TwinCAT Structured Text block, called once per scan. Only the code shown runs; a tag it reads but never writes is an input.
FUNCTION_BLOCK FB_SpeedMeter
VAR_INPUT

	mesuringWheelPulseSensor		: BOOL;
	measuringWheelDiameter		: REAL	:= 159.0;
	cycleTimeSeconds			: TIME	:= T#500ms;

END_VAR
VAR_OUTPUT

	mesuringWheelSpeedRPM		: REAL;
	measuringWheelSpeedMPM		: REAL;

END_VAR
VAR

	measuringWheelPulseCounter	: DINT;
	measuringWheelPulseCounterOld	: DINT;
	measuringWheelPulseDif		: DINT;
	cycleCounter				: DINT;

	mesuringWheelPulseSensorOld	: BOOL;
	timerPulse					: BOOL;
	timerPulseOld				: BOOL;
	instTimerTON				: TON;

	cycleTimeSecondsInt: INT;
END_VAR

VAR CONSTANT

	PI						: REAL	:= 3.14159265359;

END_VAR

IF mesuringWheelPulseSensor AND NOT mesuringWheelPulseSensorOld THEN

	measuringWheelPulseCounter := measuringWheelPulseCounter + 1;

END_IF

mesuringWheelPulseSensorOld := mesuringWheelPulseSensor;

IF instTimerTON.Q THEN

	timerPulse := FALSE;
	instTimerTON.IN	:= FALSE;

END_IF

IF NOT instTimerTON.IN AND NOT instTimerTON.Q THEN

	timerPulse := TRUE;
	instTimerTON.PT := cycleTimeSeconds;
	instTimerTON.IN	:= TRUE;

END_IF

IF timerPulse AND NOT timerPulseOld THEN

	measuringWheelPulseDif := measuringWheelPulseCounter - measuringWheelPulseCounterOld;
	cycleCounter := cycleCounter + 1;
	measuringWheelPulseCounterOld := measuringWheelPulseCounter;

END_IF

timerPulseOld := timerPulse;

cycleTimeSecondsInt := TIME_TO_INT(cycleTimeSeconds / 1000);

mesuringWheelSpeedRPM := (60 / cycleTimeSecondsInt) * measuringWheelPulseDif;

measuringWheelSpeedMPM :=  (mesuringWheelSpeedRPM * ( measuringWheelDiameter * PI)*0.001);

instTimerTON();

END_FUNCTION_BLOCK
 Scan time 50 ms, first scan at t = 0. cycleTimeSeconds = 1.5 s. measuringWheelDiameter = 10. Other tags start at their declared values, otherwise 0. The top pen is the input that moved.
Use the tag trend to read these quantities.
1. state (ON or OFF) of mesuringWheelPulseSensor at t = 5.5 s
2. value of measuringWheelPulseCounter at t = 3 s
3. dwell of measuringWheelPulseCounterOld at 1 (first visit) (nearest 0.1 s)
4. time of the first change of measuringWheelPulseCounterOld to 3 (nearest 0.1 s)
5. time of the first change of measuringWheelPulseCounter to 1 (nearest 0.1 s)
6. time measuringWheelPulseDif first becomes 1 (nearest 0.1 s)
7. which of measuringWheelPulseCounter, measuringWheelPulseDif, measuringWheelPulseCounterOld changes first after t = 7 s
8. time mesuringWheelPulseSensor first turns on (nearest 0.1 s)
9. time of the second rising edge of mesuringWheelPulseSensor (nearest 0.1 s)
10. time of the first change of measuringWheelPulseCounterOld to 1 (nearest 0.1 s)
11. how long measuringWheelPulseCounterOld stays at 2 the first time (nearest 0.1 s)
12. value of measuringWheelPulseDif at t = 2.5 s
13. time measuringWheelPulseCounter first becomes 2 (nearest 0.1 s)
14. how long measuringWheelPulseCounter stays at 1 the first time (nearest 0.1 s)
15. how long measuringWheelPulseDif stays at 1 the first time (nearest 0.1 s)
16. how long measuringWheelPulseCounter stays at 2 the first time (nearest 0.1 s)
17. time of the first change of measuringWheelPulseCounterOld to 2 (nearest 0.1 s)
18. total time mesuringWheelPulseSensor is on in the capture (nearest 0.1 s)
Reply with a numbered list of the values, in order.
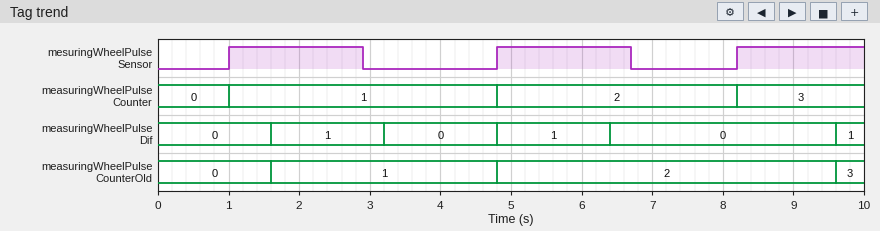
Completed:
1. ON
2. 1
3. 3.2 s
4. 9.6 s
5. 1.0 s
6. 1.6 s
7. measuringWheelPulseCounter
8. 1.0 s
9. 4.8 s
10. 1.6 s
11. 4.8 s
12. 1
13. 4.8 s
14. 3.8 s
15. 1.6 s
16. 3.4 s
17. 4.8 s
18. 5.6 s
